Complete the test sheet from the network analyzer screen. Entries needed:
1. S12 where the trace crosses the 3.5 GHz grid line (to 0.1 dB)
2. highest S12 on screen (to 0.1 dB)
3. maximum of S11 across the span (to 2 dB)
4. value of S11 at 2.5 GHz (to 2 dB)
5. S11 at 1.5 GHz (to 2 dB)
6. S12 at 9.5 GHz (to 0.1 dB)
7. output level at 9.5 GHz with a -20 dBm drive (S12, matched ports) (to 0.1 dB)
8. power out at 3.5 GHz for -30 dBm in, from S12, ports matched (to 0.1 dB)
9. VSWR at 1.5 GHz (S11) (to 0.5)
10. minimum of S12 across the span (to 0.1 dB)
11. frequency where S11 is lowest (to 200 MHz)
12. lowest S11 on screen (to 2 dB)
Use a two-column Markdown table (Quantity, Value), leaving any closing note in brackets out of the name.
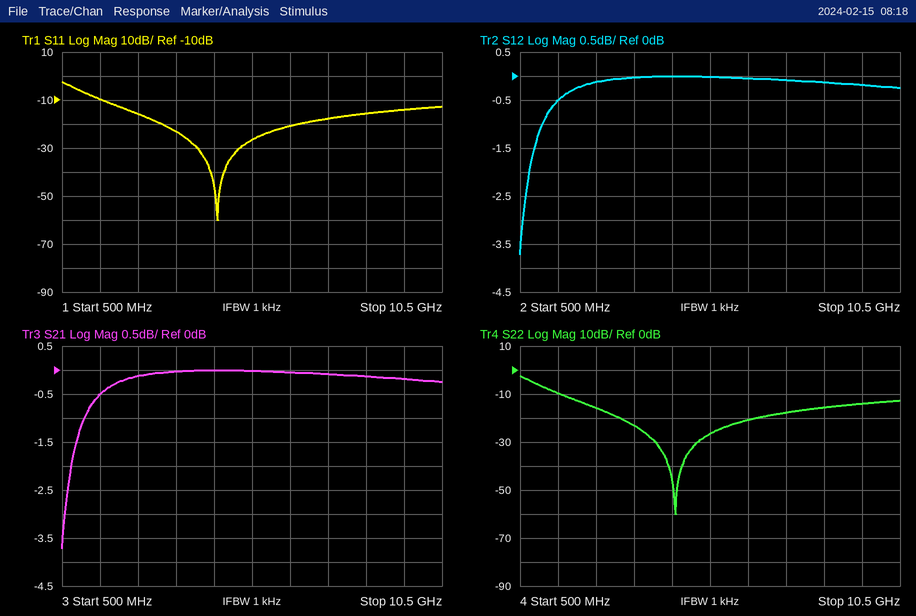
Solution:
| Quantity | Value |
|---|---|
| S12 where the trace crosses the 3.5 GHz grid line | 0.0 dB |
| highest S12 on screen | 0.0 dB |
| maximum of S11 across the span | -2 dB |
| value of S11 at 2.5 GHz | -16 dB |
| S11 at 1.5 GHz | -10 dB |
| S12 at 9.5 GHz | -0.2 dB |
| output level at 9.5 GHz with a -20 dBm drive (S12, matched ports) | -20.2 dBm |
| power out at 3.5 GHz for -30 dBm in, from S12, ports matched | -30.0 dBm |
| VSWR at 1.5 GHz (S11) | 2.0 |
| minimum of S12 across the span | -3.7 dB |
| frequency where S11 is lowest | 4.6 GHz |
| lowest S11 on screen | -60 dB |
